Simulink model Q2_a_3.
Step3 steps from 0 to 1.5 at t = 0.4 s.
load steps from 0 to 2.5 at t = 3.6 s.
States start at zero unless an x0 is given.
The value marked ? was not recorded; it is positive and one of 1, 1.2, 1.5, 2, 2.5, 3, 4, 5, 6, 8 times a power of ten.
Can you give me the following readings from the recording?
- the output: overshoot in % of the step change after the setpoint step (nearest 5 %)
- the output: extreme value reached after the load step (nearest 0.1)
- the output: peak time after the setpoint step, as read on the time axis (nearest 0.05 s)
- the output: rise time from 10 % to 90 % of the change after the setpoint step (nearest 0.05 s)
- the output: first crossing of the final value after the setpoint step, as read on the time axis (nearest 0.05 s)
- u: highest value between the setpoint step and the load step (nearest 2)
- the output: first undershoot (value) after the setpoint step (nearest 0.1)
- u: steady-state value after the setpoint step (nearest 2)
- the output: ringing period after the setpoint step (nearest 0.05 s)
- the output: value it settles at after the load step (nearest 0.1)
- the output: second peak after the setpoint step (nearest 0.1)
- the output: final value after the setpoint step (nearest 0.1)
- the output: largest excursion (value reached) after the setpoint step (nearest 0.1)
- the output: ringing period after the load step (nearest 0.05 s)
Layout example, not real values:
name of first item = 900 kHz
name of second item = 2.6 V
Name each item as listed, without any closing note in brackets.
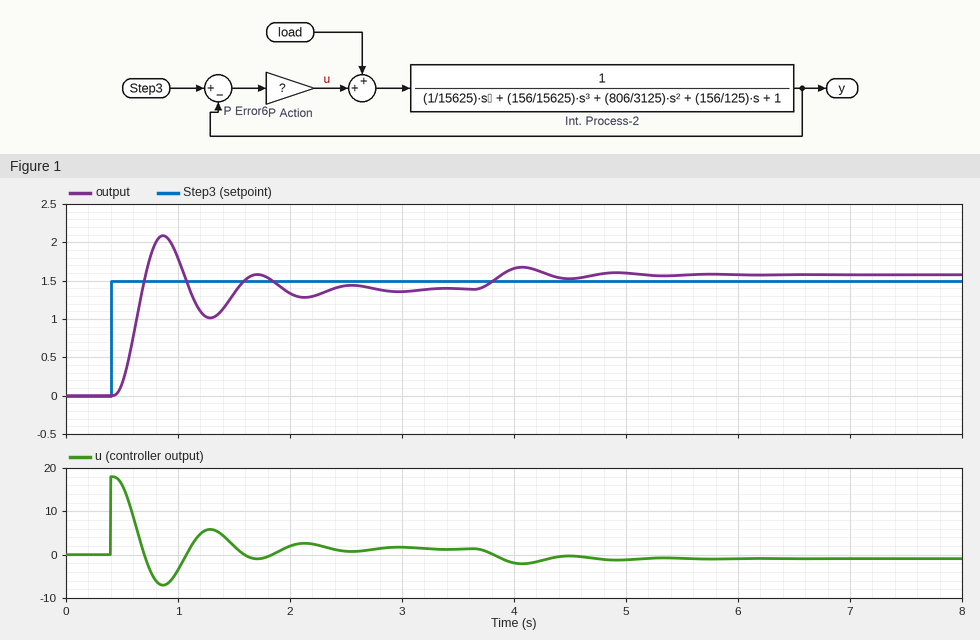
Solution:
the output: overshoot in % of the step change after the setpoint step = 50 %
the output: extreme value reached after the load step = 1.7
the output: peak time after the setpoint step, as read on the time axis = 0.85 s
the output: rise time from 10 % to 90 % of the change after the setpoint step = 0.15 s
the output: first crossing of the final value after the setpoint step, as read on the time axis = 0.70 s
u: highest value between the setpoint step and the load step = 18
the output: first undershoot (value) after the setpoint step = 1.0
u: steady-state value after the setpoint step = 2
the output: ringing period after the setpoint step = 0.85 s
the output: value it settles at after the load step = 1.6
the output: second peak after the setpoint step = 1.6
the output: final value after the setpoint step = 1.4
the output: largest excursion (value reached) after the setpoint step = 2.1
the output: ringing period after the load step = 0.85 s
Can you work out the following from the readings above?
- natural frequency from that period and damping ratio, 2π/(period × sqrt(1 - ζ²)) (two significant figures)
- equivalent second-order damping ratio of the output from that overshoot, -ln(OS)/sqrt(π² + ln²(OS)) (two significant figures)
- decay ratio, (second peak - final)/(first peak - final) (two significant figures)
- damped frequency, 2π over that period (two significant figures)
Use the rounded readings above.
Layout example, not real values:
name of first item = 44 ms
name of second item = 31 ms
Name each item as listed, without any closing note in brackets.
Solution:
natural frequency from that period and damping ratio, 2π/(period × sqrt(1 - ζ²)) = 7.6 rad/s
equivalent second-order damping ratio of the output from that overshoot, -ln(OS)/sqrt(π² + ln²(OS)) = 0.22
decay ratio, (second peak - final)/(first peak - final) = 0.29
damped frequency, 2π over that period = 7.4 rad/s
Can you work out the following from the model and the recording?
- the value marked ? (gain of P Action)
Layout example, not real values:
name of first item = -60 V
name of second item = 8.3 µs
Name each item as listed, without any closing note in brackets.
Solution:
the value marked ? = 12
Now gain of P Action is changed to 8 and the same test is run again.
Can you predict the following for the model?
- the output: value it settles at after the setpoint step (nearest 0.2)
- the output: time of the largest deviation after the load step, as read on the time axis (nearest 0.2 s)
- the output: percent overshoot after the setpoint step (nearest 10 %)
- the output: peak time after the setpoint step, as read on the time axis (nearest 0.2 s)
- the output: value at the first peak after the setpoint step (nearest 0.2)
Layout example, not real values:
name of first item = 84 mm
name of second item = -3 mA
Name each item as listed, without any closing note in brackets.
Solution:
the output: value it settles at after the setpoint step = 1.4
the output: time of the largest deviation after the load step, as read on the time axis = 4.2 s
the output: percent overshoot after the setpoint step = 40 %
the output: peak time after the setpoint step, as read on the time axis = 1.0 s
the output: value at the first peak after the setpoint step = 1.8
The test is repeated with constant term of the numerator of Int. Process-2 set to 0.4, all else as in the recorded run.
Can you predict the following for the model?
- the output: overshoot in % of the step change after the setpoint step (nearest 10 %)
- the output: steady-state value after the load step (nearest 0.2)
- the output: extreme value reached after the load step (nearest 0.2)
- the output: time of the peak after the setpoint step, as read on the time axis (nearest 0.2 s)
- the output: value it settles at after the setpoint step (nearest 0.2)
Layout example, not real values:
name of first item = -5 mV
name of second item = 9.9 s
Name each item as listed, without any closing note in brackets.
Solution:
the output: overshoot in % of the step change after the setpoint step = 20 %
the output: steady-state value after the load step = 1.4
the output: extreme value reached after the load step = 1.4
the output: time of the peak after the setpoint step, as read on the time axis = 1.2 s
the output: value it settles at after the setpoint step = 1.2
